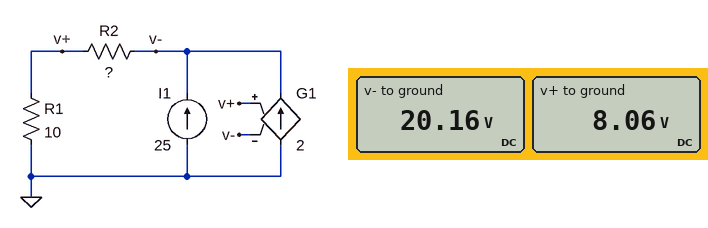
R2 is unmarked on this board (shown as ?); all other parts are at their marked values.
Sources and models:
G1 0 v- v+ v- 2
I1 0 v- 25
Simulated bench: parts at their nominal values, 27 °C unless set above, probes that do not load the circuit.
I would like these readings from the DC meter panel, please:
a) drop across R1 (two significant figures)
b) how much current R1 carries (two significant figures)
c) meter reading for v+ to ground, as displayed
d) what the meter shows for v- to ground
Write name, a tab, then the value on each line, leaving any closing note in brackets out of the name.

drop across R1	8.1 V
how much current R1 carries	810 mA
meter reading for v+ to ground, as displayed	8.06 V
what the meter shows for v- to ground	20.16 V
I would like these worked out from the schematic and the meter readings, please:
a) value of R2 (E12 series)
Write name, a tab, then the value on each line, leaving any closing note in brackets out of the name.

value of R2	15 Ω
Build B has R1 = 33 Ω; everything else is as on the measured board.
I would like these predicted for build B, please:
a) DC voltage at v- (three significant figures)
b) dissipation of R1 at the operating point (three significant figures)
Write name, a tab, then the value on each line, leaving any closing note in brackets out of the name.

DC voltage at v-	38.7 V
dissipation of R1 at the operating point	21.5 W
